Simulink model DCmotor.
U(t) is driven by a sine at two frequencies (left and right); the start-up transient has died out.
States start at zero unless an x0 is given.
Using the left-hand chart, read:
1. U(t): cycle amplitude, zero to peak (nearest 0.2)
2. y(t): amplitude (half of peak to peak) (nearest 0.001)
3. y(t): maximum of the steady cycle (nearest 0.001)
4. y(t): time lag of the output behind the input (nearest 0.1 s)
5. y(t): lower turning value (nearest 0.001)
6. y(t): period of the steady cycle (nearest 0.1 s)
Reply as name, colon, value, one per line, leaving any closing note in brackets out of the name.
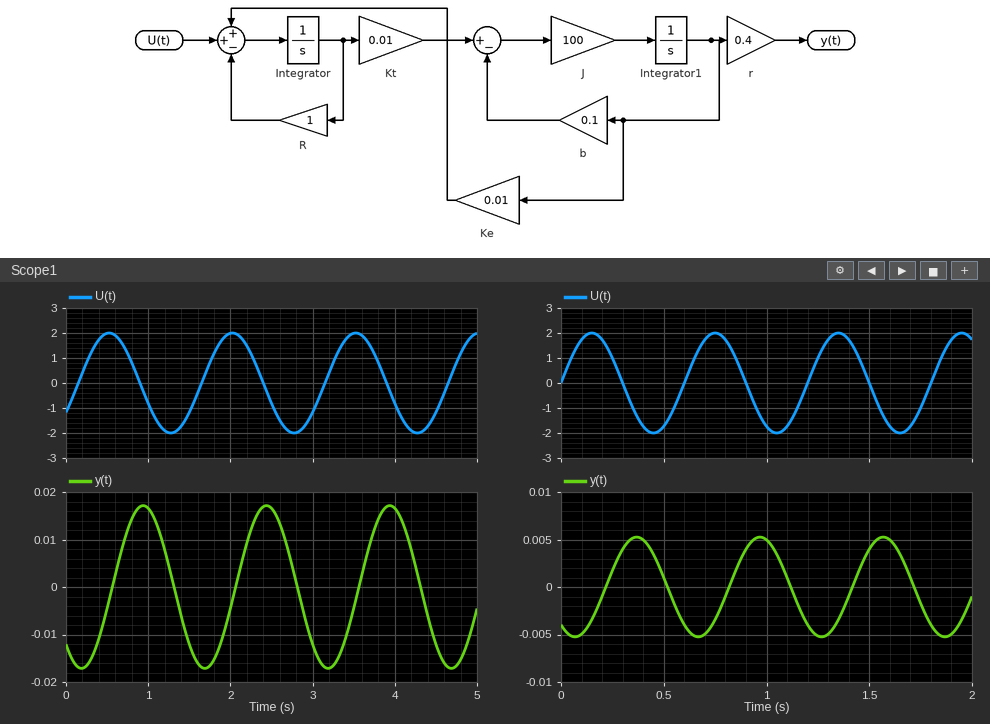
U(t): cycle amplitude, zero to peak: 2.0
y(t): amplitude (half of peak to peak): 0.017
y(t): maximum of the steady cycle: 0.017
y(t): time lag of the output behind the input: 0.4 s
y(t): lower turning value: -0.017
y(t): period of the steady cycle: 1.5 s
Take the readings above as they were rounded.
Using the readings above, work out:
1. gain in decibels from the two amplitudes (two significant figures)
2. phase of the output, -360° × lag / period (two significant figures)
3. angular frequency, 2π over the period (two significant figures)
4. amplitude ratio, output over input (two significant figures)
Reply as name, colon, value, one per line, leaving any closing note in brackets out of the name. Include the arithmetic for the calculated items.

gain in decibels from the two amplitudes: 20 log10(0.017 / 2) = -41 dB
phase of the output, -360° × lag / period: -360 × 0.4 / 1.5 = -96°
angular frequency, 2π over the period: 2π / 1.5 = 4.2 rad/s
amplitude ratio, output over input: 0.017 / 2 = 0.0085
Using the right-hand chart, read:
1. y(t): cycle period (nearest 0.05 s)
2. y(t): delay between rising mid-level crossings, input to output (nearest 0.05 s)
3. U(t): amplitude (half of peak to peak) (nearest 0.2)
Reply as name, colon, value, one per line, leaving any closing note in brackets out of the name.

y(t): cycle period: 0.60 s
y(t): delay between rising mid-level crossings, input to output: 0.20 s
U(t): amplitude (half of peak to peak): 2.0
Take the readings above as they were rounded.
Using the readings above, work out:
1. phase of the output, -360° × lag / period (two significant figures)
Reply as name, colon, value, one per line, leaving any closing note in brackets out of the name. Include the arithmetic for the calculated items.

phase of the output, -360° × lag / period: -360 × 0.2 / 0.6 = -120°
